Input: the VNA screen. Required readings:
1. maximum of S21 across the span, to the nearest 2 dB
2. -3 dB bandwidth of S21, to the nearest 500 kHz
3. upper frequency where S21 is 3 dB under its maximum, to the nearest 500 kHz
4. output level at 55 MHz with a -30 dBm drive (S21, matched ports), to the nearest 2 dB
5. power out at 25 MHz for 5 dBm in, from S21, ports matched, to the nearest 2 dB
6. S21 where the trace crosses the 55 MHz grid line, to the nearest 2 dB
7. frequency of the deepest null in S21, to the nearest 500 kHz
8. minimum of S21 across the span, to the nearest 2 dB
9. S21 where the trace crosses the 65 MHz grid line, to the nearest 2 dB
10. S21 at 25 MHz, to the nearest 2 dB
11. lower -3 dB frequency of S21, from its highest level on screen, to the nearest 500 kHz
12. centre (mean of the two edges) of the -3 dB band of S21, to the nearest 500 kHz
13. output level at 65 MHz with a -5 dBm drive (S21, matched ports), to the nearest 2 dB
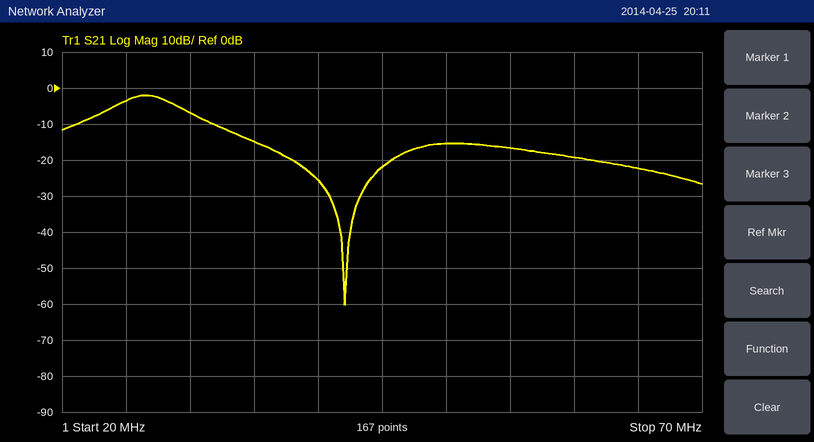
-2 dB
5.0 MHz
29.0 MHz
-46 dBm
2 dBm
-16 dB
42.0 MHz
-60 dB
-22 dB
-4 dB
24.0 MHz
26.5 MHz
-28 dBm
